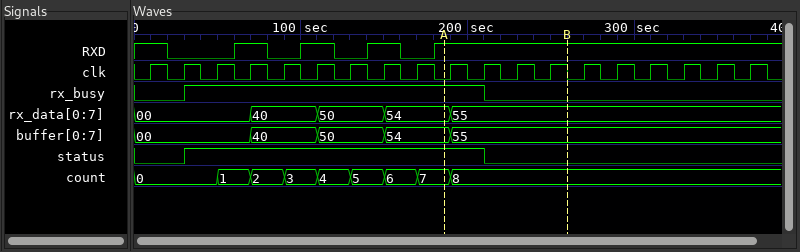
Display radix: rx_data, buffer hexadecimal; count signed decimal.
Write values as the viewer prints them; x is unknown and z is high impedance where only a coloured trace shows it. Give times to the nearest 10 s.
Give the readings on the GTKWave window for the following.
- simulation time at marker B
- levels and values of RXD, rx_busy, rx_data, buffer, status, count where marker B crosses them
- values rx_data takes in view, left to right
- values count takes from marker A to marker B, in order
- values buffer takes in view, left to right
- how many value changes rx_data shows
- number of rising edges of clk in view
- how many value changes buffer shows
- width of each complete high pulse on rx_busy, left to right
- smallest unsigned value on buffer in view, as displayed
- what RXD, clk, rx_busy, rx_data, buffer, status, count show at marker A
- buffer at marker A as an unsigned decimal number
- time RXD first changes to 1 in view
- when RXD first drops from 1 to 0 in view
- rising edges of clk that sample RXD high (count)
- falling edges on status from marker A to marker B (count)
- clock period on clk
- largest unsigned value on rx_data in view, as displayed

260 s
RXD=1, rx_busy=0, rx_data=55, buffer=55, status=0, count=8
00, 40, 50, 54, 55
7, 8
00, 40, 50, 54, 55
4
19
4
180 s
00
RXD=1, clk=0, rx_busy=1, rx_data=54, buffer=54, status=1, count=7
84
60 s
20 s
14
1
20 s
55
